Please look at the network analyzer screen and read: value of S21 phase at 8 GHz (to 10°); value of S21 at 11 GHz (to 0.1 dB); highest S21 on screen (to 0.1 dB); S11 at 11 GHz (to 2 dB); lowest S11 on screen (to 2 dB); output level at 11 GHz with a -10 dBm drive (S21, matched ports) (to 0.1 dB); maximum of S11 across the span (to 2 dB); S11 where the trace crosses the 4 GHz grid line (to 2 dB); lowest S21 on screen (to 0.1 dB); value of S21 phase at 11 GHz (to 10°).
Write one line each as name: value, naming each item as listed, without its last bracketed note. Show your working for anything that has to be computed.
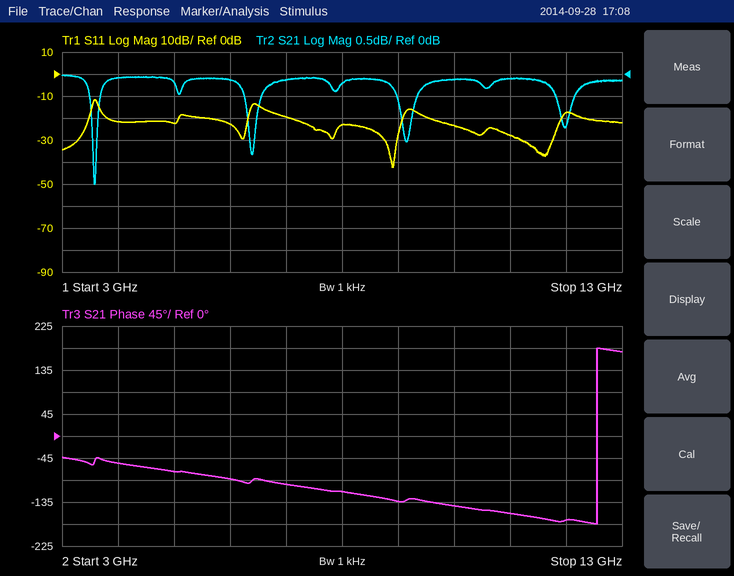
value of S21 phase at 8 GHz: -110°
value of S21 at 11 GHz: -0.1 dB
highest S21 on screen: 0.0 dB
S11 at 11 GHz: -28 dB
lowest S11 on screen: -42 dB
output level at 11 GHz with a -10 dBm drive (S21, matched ports): -10 dBm + (-0.1 dB) = -10.1 dBm
maximum of S11 across the span: -12 dB
S11 where the trace crosses the 4 GHz grid line: -22 dB
lowest S21 on screen: -2.5 dB
value of S21 phase at 11 GHz: -160°
